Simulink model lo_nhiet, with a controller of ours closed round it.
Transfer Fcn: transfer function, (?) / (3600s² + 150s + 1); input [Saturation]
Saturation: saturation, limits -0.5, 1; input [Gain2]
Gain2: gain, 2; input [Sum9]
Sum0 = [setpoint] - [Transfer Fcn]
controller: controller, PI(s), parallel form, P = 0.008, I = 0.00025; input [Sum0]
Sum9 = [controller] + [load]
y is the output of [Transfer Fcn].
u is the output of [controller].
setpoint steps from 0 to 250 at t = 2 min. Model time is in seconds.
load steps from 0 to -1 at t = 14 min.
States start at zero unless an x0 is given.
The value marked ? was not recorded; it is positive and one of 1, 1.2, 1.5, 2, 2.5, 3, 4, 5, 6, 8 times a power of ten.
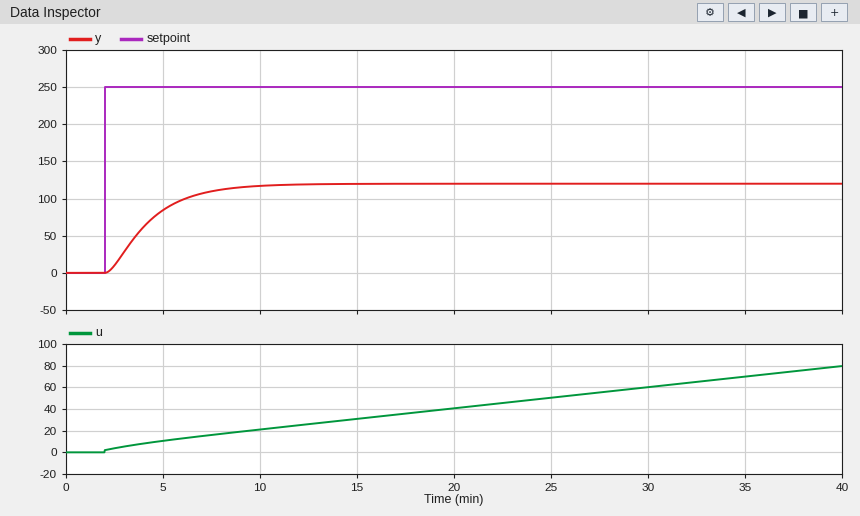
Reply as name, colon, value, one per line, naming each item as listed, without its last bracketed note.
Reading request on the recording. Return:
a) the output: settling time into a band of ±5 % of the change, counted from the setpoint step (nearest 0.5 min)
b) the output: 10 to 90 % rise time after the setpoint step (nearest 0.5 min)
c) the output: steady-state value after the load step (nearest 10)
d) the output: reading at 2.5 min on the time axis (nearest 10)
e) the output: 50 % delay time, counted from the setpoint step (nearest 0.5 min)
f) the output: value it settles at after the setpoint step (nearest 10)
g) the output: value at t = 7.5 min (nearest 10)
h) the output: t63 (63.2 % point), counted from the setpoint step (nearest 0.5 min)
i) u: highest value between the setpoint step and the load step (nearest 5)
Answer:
the output: settling time into a band of ±5 % of the change, counted from the setpoint step: 6.5 min
the output: 10 to 90 % rise time after the setpoint step: 4.5 min
the output: steady-state value after the load step: 120
the output: reading at 2.5 min on the time axis: 10
the output: 50 % delay time, counted from the setpoint step: 2.0 min
the output: value it settles at after the setpoint step: 120
the output: value at t = 7.5 min: 110
the output: t63 (63.2 % point), counted from the setpoint step: 2.5 min
u: highest value between the setpoint step and the load step: 30
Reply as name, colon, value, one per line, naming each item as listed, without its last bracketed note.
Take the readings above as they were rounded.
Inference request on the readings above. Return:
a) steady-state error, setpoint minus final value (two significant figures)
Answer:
steady-state error, setpoint minus final value: 130
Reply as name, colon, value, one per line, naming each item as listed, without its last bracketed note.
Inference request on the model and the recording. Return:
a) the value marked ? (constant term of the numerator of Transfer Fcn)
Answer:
the value marked ?: 120
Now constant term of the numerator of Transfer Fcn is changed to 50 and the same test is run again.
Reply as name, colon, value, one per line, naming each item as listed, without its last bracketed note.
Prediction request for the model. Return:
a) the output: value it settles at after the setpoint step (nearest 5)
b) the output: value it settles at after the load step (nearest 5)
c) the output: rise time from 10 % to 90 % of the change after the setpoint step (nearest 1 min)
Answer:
the output: value it settles at after the setpoint step: 50
the output: value it settles at after the load step: 50
the output: rise time from 10 % to 90 % of the change after the setpoint step: 5 min
